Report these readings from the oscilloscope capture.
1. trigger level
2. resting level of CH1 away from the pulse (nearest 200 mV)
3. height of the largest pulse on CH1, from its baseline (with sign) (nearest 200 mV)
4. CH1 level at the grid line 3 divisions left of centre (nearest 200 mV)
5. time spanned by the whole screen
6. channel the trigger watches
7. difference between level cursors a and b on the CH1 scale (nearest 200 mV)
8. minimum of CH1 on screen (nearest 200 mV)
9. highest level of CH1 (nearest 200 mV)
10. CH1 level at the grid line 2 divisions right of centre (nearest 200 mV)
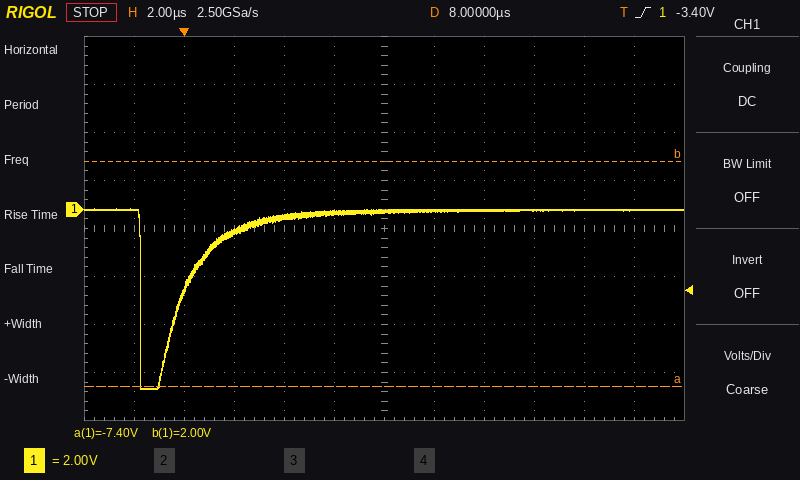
-3.40 V
0.0 V
-7.4 V
-1.0 V
24 µs
CH1
9.4 V
-7.4 V
0.0 V
0.0 V
